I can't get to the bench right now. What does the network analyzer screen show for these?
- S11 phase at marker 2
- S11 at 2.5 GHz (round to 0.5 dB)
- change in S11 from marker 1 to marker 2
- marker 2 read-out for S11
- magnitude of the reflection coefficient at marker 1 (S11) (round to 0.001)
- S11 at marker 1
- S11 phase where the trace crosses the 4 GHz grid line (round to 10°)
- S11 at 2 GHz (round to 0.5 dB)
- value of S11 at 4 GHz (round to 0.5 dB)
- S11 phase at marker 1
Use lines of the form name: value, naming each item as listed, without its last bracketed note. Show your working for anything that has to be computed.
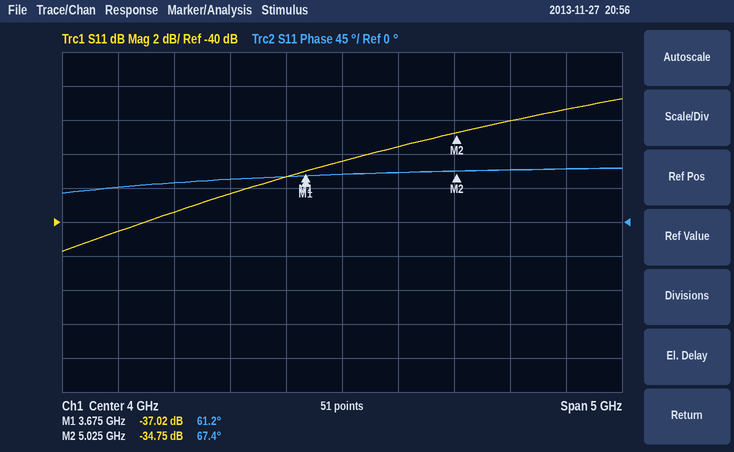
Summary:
S11 phase at marker 2: 67.4°
S11 at 2.5 GHz: -39.5 dB
change in S11 from marker 1 to marker 2: -34.75 − (-37.02) = 2.27 dB
marker 2 read-out for S11: -34.75 dB
magnitude of the reflection coefficient at marker 1 (S11): 10^(-37.02/20) ≈ 0.014
S11 at marker 1: -37.02 dB
S11 phase where the trace crosses the 4 GHz grid line: 60°
S11 at 2 GHz: -40.5 dB
value of S11 at 4 GHz: -36.5 dB
S11 phase at marker 1: 61.2°
